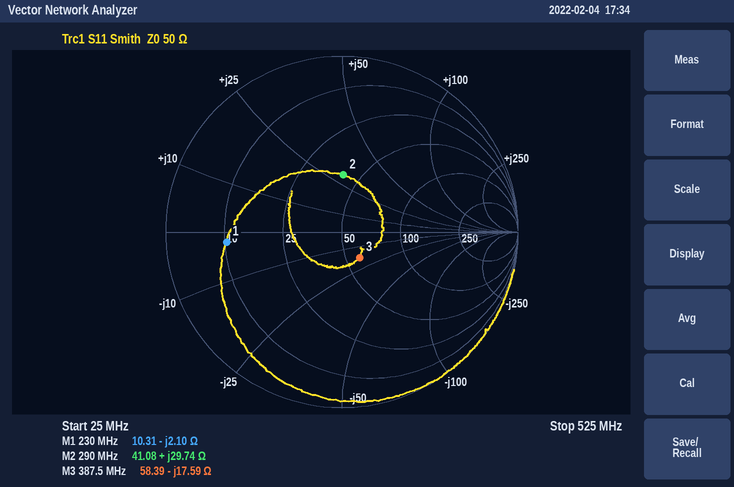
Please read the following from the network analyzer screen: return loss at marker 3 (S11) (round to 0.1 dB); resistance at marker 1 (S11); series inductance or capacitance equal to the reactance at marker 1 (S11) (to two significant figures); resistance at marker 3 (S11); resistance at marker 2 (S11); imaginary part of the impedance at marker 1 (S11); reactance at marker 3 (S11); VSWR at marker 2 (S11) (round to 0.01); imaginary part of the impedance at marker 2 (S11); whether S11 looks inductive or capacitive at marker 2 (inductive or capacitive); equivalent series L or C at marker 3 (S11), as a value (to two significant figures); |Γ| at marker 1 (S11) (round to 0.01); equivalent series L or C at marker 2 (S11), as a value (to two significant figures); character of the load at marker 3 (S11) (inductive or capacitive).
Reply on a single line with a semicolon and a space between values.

15.0 dB; 10.31 Ω; 330 pF; 58.39 Ω; 41.08 Ω; -2.10 Ω; -17.59 Ω; 1.96; +29.74 Ω; inductive; 23 pF; 0.66; 16 nH; capacitive
